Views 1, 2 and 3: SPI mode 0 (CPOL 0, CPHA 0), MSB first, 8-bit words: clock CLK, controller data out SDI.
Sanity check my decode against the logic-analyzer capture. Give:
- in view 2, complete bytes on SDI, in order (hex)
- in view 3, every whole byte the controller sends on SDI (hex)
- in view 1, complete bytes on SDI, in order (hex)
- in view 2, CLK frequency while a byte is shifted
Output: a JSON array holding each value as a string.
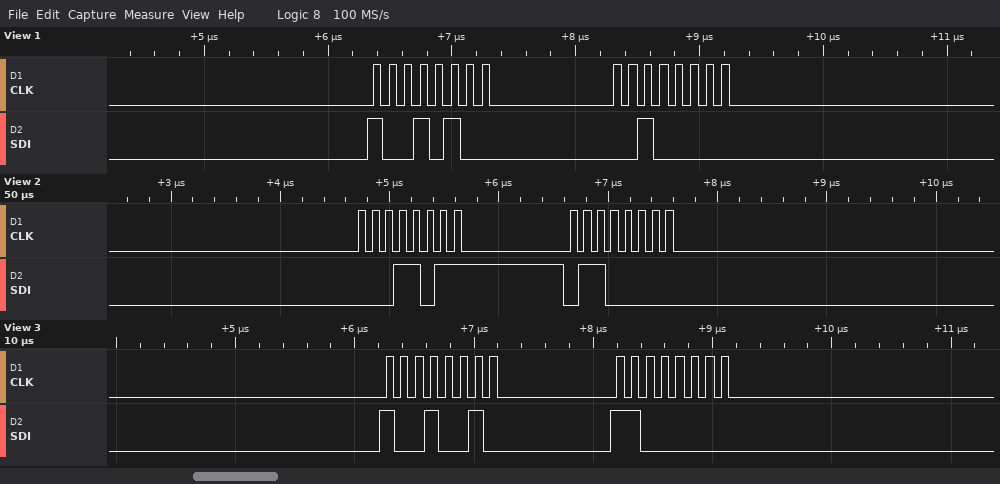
["1B 60", "92 C0", "0x94 0x20", "8 MHz"]
